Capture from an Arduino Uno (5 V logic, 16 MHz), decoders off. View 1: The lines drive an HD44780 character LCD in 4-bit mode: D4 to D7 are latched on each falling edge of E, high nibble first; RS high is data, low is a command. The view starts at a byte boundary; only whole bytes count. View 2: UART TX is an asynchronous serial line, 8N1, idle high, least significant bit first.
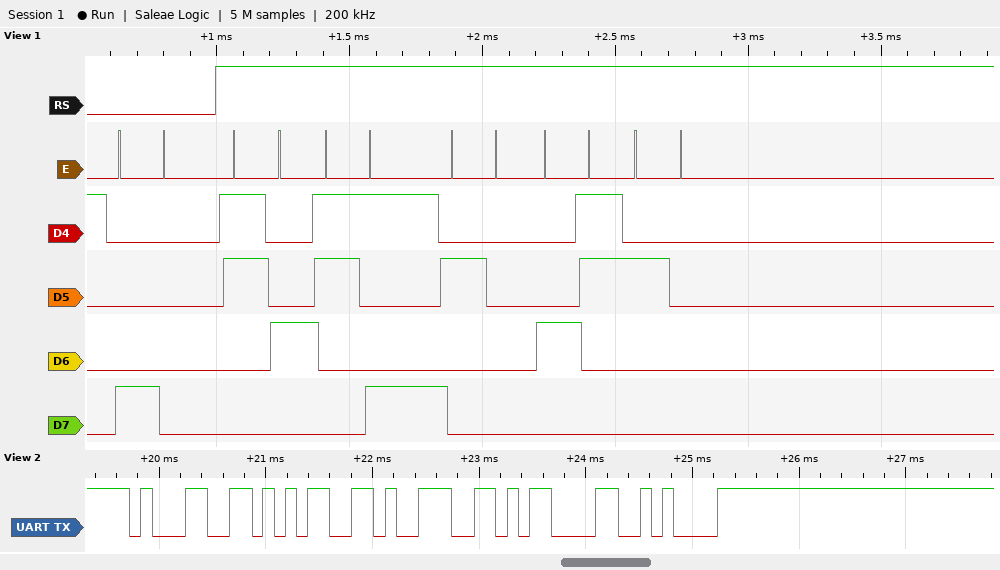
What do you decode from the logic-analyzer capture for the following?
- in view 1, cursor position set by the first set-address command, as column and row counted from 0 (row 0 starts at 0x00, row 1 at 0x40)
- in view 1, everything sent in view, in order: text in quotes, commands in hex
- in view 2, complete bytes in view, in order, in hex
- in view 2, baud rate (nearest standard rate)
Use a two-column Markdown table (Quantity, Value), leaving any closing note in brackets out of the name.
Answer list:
| Quantity | Value |
|---|---|
| in view 1, cursor position set by the first set-address command, as column and row counted from 0 | column 0, row 0 |
| in view 1, everything sent in view, in order: text in quotes, commands in hex | 0x80 "49 C " |
| in view 2, complete bytes in view, in order, in hex | 31 35 39 0D 0A |
| in view 2, baud rate | 9600 baud |
